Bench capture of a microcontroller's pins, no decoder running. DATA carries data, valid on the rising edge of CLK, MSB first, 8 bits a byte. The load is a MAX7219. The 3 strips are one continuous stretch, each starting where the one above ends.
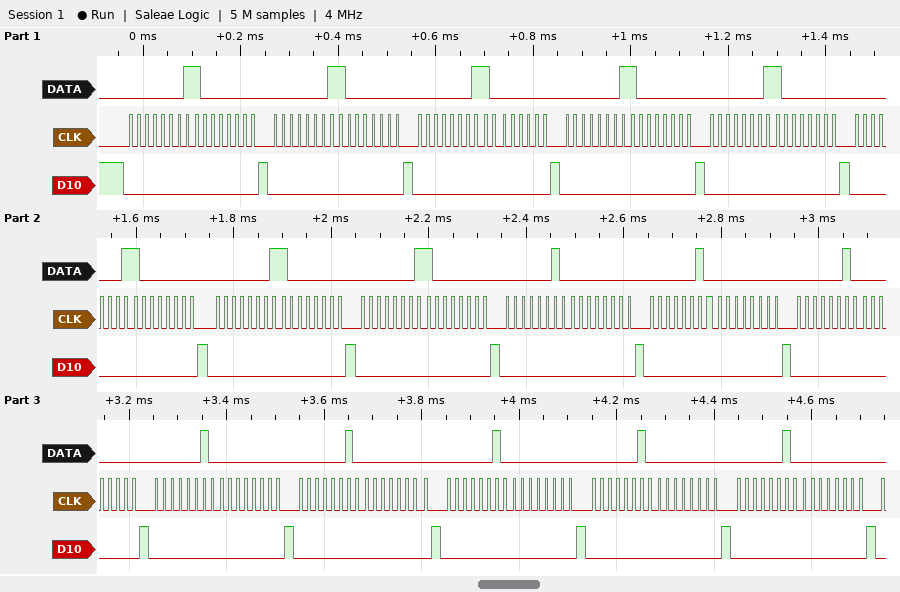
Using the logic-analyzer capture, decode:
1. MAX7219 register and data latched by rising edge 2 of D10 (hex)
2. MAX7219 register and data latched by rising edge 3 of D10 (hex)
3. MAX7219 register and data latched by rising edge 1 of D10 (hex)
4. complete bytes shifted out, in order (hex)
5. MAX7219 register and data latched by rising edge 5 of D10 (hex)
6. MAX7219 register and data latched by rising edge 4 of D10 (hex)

register 0x1, data 0x80
register 0x1, data 0x80
register 0x1, data 0x80
0x01 0x80 0x01 0x80 0x01 0x80 0x01 0x80 0x01 0x80 0x01 0x80 0x01 0x80 0x01 0x80 0x02 0x00 0x02 0x00 0x02 0x00 0x02 0x00 0x02 0x00 0x02 0x00 0x02 0x00 0x02 0x00
register 0x1, data 0x80
register 0x1, data 0x80
